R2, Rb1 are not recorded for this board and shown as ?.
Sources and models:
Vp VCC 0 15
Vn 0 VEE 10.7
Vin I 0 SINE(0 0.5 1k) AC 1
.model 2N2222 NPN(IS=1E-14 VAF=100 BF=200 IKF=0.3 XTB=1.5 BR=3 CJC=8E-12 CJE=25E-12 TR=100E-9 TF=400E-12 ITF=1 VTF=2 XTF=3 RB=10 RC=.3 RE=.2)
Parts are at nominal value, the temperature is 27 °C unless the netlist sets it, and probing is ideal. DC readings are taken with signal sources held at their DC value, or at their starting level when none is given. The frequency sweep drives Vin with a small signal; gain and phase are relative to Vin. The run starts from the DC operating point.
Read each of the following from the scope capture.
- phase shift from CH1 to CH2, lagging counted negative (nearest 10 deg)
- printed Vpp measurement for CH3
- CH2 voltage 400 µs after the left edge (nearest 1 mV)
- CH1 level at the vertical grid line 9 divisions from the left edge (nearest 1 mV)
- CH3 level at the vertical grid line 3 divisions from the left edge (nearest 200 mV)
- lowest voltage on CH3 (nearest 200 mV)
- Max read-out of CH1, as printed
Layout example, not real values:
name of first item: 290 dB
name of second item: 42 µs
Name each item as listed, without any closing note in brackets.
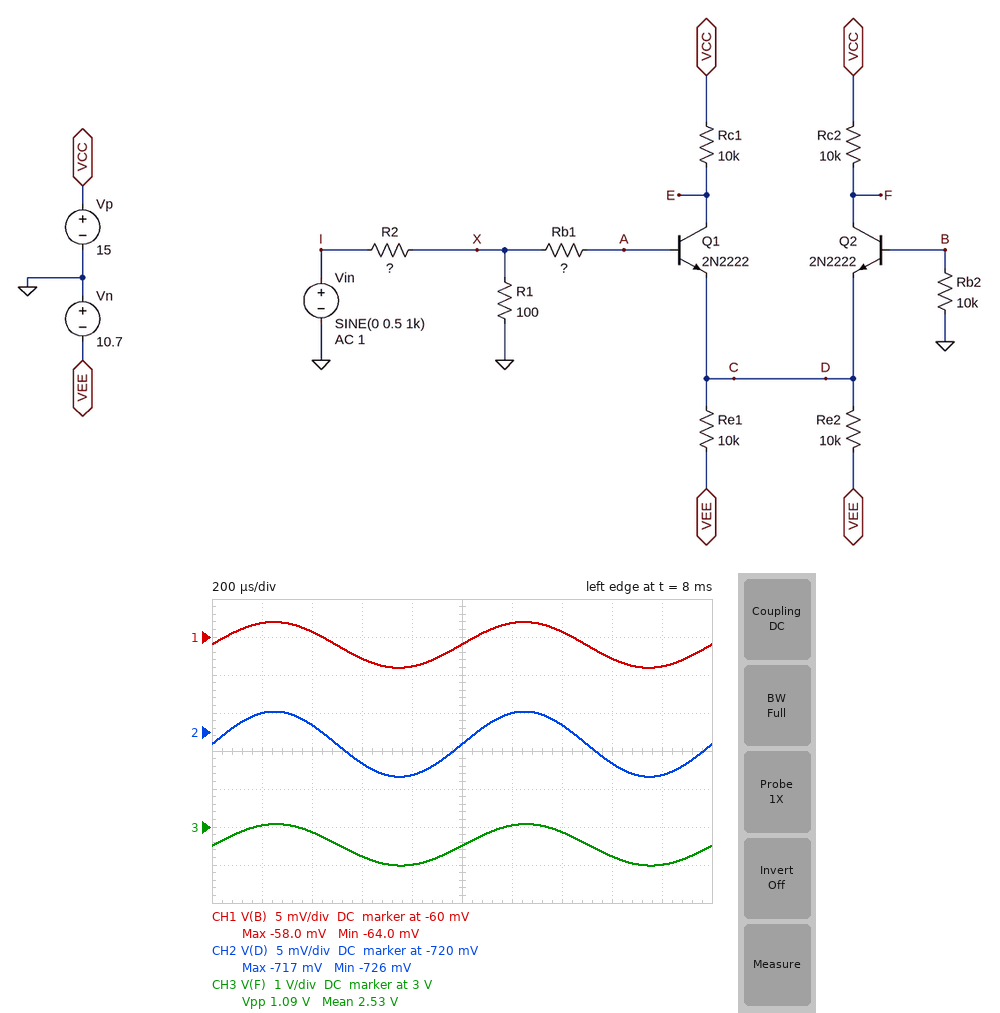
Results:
phase shift from CH1 to CH2, lagging counted negative: 0 deg
printed Vpp measurement for CH3: 1.09 V
CH2 voltage 400 µs after the left edge: -719 mV
CH1 level at the vertical grid line 9 divisions from the left edge: -64 mV
CH3 level at the vertical grid line 3 divisions from the left edge: 2.2 V
lowest voltage on CH3: 2.0 V
Max read-out of CH1, as printed: -58.0 mV
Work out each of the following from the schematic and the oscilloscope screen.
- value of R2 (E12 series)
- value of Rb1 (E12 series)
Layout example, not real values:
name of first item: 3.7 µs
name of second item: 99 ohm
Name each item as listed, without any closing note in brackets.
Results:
value of R2: 3.9 kΩ
value of Rb1: 22 kΩ
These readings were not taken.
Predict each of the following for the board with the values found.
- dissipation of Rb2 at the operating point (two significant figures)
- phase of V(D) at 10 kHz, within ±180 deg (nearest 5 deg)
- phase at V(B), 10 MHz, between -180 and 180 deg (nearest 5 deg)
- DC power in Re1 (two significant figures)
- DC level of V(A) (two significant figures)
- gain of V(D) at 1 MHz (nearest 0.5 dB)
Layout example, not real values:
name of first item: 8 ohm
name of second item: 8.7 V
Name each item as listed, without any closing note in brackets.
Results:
dissipation of Rb2 at the operating point: 370 nW
phase of V(D) at 10 kHz, within ±180 deg: 0 deg
phase at V(B), 10 MHz, between -180 and 180 deg: -20 deg
DC power in Re1: 10 mW
DC level of V(A): -76 mV
gain of V(D) at 1 MHz: -43.5 dB
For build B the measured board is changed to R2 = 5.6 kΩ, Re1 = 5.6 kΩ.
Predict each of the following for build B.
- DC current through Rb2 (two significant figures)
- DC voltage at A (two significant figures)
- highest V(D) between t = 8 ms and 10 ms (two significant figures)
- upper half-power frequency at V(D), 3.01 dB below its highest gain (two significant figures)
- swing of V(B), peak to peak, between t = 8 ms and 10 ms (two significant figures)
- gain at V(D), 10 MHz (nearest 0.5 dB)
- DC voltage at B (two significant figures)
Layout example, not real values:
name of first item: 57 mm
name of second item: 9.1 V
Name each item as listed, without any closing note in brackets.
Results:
DC current through Rb2: 12 µA
DC voltage at A: -130 mV
highest V(D) between t = 8 ms and 10 ms: -780 mV
upper half-power frequency at V(D), 3.01 dB below its highest gain: 240 kHz
swing of V(B), peak to peak, between t = 8 ms and 10 ms: 16 mV
gain at V(D), 10 MHz: -57.5 dB
DC voltage at B: -120 mV
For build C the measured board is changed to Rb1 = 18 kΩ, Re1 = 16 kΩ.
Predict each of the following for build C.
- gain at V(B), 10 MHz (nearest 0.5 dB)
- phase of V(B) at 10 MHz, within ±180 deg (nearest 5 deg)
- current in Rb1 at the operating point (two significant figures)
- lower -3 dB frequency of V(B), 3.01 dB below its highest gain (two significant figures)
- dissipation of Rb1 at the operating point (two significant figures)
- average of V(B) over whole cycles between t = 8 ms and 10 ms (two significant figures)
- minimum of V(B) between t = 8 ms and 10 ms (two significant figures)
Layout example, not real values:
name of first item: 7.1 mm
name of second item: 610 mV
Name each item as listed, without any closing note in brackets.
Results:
gain at V(B), 10 MHz: -51.0 dB
phase of V(B) at 10 MHz, within ±180 deg: -15 deg
current in Rb1 at the operating point: 3.1 µA
lower -3 dB frequency of V(B), 3.01 dB below its highest gain: 11 kHz
dissipation of Rb1 at the operating point: 170 nW
average of V(B) over whole cycles between t = 8 ms and 10 ms: -45 mV
minimum of V(B) between t = 8 ms and 10 ms: -48 mV
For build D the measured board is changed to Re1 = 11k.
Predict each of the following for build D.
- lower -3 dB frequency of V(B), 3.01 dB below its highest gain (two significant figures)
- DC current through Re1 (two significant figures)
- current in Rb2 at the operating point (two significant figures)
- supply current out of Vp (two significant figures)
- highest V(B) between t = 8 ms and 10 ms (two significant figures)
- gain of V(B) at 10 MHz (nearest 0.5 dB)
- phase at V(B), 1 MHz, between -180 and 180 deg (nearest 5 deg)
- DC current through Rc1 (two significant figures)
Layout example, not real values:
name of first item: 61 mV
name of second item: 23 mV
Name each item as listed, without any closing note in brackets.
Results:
lower -3 dB frequency of V(B), 3.01 dB below its highest gain: 8.4 kHz
DC current through Re1: 910 µA
current in Rb2 at the operating point: 5.8 µA
supply current out of Vp: 1.9 mA
highest V(B) between t = 8 ms and 10 ms: -55 mV
gain of V(B) at 10 MHz: -53.0 dB
phase at V(B), 1 MHz, between -180 and 180 deg: -30 deg
DC current through Rc1: 710 µA
